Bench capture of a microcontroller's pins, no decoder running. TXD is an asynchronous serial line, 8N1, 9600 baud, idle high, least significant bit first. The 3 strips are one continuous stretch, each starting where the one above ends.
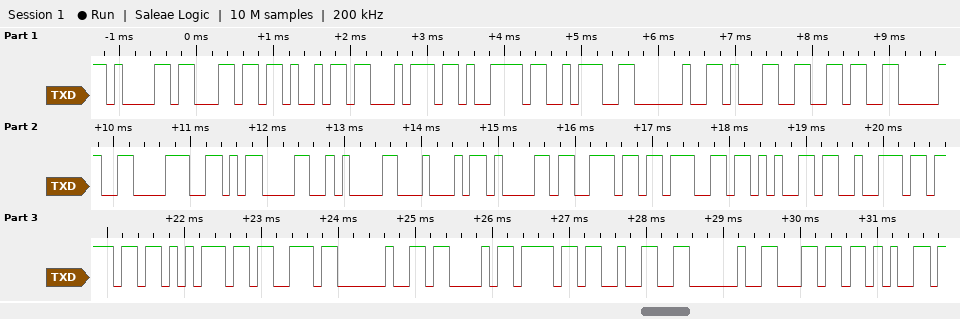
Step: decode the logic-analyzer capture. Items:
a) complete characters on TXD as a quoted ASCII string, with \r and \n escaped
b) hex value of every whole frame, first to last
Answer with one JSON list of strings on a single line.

["\"ality: 1608\\r\\nDangerous Co2 le\"", "0x61 0x6C 0x69 0x74 0x79 0x3A 0x20 0x31 0x36 0x30 0x38 0x0D 0x0A 0x44 0x61 0x6E 0x67 0x65 0x72 0x6F 0x75 0x73 0x20 0x43 0x6F 0x32 0x20 0x6C 0x65"]
